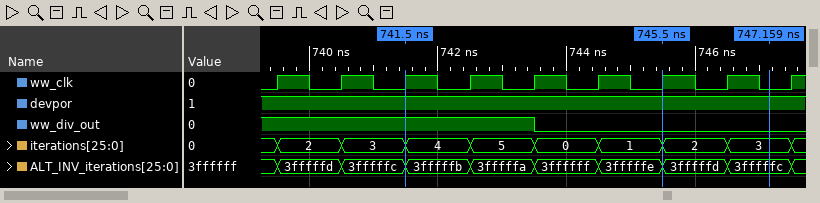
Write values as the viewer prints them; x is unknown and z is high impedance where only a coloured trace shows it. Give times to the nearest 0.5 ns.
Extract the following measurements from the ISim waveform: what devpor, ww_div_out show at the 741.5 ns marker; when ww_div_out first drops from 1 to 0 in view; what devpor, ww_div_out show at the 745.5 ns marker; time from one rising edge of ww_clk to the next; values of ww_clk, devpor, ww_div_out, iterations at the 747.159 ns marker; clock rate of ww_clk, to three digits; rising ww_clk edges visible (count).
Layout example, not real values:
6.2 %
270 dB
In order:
devpor=1, ww_div_out=1
743.5 ns
devpor=1, ww_div_out=0
1 ns
ww_clk=0, devpor=1, ww_div_out=0, iterations=3
1.00 GHz
9
